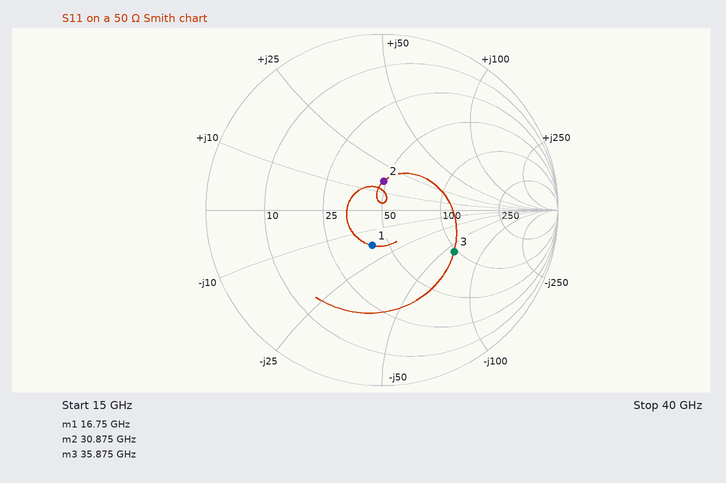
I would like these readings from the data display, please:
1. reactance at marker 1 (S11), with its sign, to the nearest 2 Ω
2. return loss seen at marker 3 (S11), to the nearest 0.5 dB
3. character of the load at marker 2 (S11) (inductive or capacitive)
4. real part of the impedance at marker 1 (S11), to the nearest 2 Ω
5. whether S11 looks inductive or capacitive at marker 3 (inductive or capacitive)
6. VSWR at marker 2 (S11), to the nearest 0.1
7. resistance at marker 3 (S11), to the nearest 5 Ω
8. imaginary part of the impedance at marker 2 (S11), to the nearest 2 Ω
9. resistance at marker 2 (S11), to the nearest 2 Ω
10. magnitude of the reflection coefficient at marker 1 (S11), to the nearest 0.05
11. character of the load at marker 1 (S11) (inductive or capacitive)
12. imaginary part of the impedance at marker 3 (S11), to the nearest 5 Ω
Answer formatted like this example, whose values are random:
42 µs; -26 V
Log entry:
-18 Ω; 6.5 dB; inductive; 42 Ω; capacitive; 1.4; 95 Ω; +16 Ω; 48 Ω; 0.20; capacitive; -60 Ω
